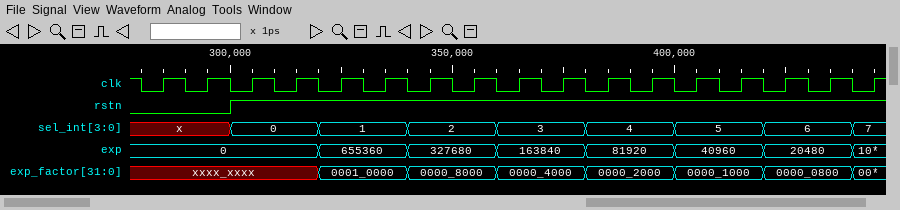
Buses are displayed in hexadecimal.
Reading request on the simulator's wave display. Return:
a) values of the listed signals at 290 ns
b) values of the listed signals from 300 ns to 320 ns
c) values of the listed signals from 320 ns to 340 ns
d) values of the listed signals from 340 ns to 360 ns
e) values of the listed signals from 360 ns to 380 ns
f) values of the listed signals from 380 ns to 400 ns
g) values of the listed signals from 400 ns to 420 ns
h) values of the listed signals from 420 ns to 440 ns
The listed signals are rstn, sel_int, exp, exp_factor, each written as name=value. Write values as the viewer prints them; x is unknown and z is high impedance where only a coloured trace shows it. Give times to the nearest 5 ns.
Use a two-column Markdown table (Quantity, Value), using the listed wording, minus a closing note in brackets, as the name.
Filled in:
| Quantity | Value |
|---|---|
| values of the listed signals at 290 ns | rstn=0, sel_int=x, exp=0, exp_factor=xxxx_xxxx |
| values of the listed signals from 300 ns to 320 ns | rstn=1, sel_int=0, exp=0, exp_factor=xxxx_xxxx |
| values of the listed signals from 320 ns to 340 ns | rstn=1, sel_int=1, exp=655360, exp_factor=0001_0000 |
| values of the listed signals from 340 ns to 360 ns | rstn=1, sel_int=2, exp=327680, exp_factor=0000_8000 |
| values of the listed signals from 360 ns to 380 ns | rstn=1, sel_int=3, exp=163840, exp_factor=0000_4000 |
| values of the listed signals from 380 ns to 400 ns | rstn=1, sel_int=4, exp=81920, exp_factor=0000_2000 |
| values of the listed signals from 400 ns to 420 ns | rstn=1, sel_int=5, exp=40960, exp_factor=0000_1000 |
| values of the listed signals from 420 ns to 440 ns | rstn=1, sel_int=6, exp=20480, exp_factor=0000_0800 |
